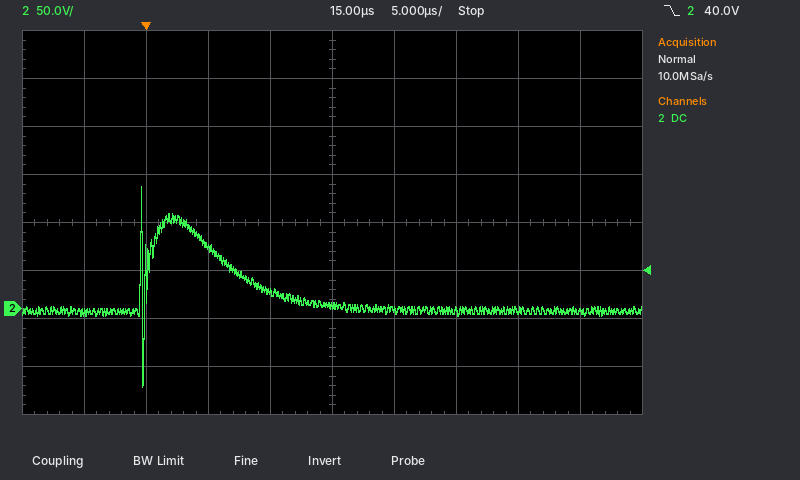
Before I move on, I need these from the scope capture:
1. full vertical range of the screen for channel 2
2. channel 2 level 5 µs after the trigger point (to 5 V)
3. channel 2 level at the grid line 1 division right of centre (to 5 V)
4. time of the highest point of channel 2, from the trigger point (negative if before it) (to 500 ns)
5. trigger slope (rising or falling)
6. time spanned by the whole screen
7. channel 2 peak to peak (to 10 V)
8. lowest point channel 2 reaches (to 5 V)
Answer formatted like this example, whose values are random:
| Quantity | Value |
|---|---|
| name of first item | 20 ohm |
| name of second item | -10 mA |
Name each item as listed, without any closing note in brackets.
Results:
| Quantity | Value |
|---|---|
| full vertical range of the screen for channel 2 | 400 V |
| channel 2 level 5 µs after the trigger point | 65 V |
| channel 2 level at the grid line 1 division right of centre | 0 V |
| time of the highest point of channel 2, from the trigger point (negative if before it) | -500 ns |
| trigger slope | falling |
| time spanned by the whole screen | 50 µs |
| channel 2 peak to peak | 210 V |
| lowest point channel 2 reaches | -80 V |
